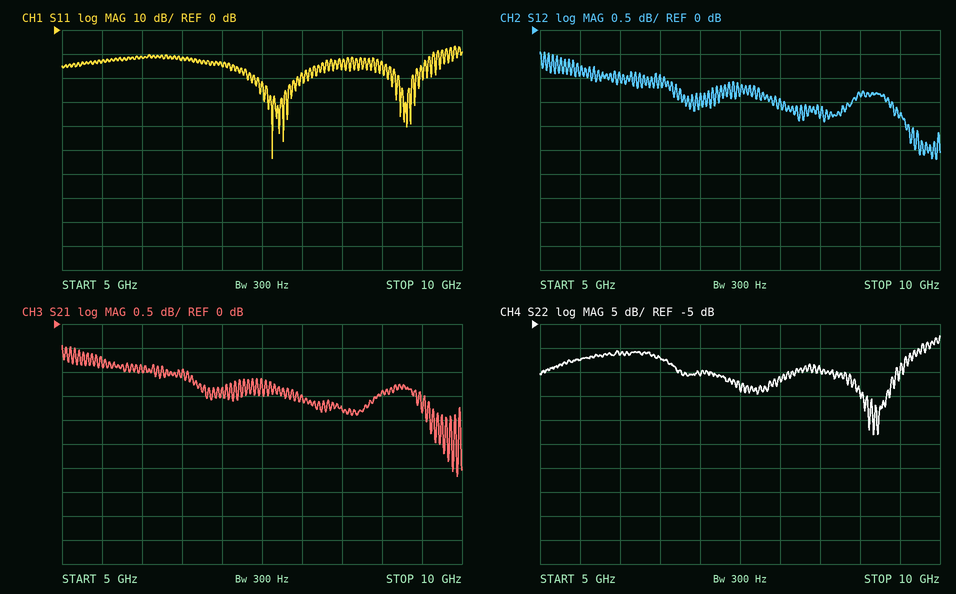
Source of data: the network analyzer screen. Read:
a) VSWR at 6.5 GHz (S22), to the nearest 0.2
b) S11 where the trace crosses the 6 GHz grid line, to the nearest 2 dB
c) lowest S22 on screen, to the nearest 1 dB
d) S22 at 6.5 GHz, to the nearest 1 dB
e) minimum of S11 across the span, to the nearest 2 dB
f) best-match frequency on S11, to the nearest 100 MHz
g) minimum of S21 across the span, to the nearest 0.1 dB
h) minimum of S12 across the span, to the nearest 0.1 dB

1.6
-12 dB
-28 dB
-12 dB
-54 dB
7.6 GHz
-3.2 dB
-2.7 dB
